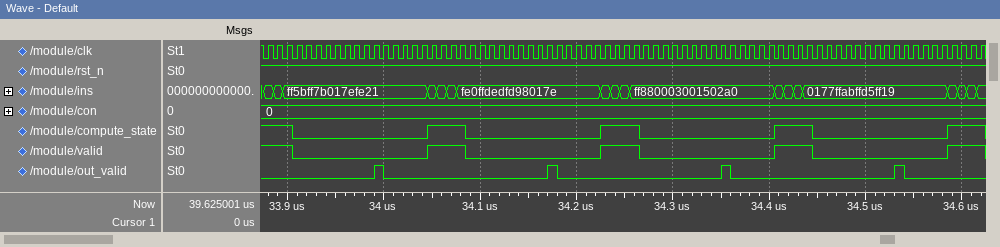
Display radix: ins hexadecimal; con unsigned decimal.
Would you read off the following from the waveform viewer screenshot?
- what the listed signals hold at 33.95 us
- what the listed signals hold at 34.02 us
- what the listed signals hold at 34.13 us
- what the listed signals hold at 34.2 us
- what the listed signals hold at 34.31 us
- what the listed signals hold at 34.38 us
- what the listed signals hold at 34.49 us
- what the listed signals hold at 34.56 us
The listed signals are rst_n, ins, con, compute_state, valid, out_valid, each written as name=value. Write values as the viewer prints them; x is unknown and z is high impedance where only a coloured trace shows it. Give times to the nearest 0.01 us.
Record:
rst_n=1, ins=ff5bff7b017efe21, con=0, compute_state=0, valid=0, out_valid=0
rst_n=1, ins=ff5bff7b017efe21, con=0, compute_state=0, valid=0, out_valid=0
rst_n=1, ins=fe0ffdedfd98017e, con=0, compute_state=0, valid=0, out_valid=0
rst_n=1, ins=fe0ffdedfd98017e, con=0, compute_state=0, valid=0, out_valid=0
rst_n=1, ins=ff880003001502a0, con=0, compute_state=0, valid=0, out_valid=0
rst_n=1, ins=ff880003001502a0, con=0, compute_state=0, valid=0, out_valid=0
rst_n=1, ins=0177ffabffd5ff19, con=0, compute_state=0, valid=0, out_valid=0
rst_n=1, ins=0177ffabffd5ff19, con=0, compute_state=0, valid=0, out_valid=0
